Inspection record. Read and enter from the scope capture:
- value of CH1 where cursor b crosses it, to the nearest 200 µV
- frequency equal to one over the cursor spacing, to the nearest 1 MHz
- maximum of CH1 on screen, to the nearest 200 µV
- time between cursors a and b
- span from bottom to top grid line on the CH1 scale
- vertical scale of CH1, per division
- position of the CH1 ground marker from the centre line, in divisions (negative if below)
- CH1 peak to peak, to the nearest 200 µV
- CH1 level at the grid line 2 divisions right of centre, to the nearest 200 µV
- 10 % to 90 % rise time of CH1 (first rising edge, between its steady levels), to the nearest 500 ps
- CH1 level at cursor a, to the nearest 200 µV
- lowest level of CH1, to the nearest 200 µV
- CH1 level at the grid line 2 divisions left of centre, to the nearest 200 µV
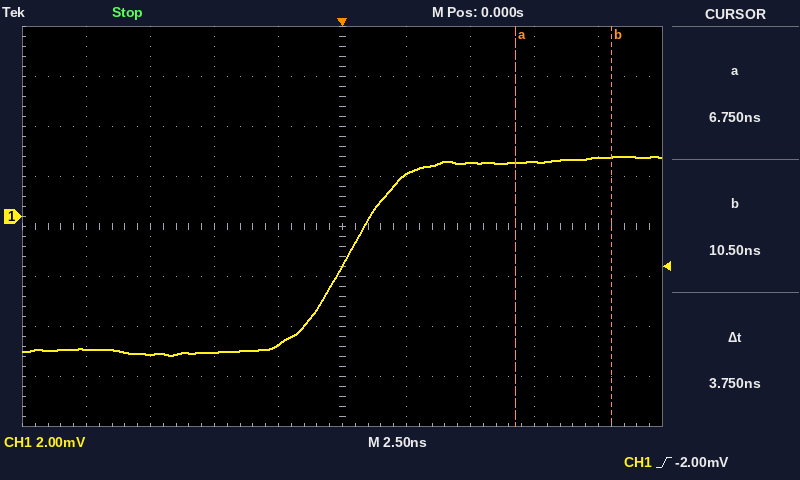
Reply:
2.4 mV
267 MHz
2.4 mV
3.75 ns
16 mV
2 mV
+0.2 div
8.0 mV
2.2 mV
4.0 ns
2.2 mV
-5.6 mV
-5.4 mV
